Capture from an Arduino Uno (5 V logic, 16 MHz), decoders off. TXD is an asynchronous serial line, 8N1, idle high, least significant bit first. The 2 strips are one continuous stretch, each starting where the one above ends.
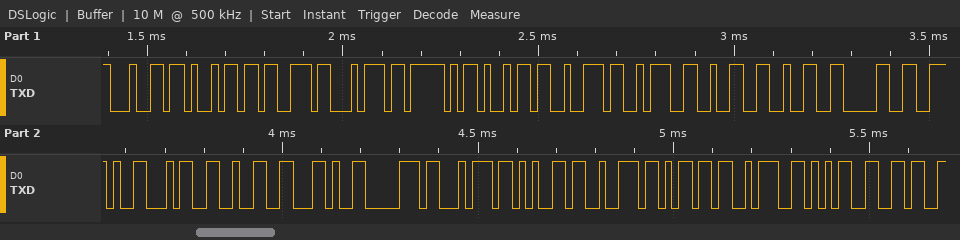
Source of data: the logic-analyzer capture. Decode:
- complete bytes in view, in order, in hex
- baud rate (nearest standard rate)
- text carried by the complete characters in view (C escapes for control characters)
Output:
64 69 73 74 5F 69 72 3A 32 32 30 2E 34 32 2C 70 74 65 72 6D 3A 35 36
57600 baud
"dist_ir:220.42,pterm:56"
